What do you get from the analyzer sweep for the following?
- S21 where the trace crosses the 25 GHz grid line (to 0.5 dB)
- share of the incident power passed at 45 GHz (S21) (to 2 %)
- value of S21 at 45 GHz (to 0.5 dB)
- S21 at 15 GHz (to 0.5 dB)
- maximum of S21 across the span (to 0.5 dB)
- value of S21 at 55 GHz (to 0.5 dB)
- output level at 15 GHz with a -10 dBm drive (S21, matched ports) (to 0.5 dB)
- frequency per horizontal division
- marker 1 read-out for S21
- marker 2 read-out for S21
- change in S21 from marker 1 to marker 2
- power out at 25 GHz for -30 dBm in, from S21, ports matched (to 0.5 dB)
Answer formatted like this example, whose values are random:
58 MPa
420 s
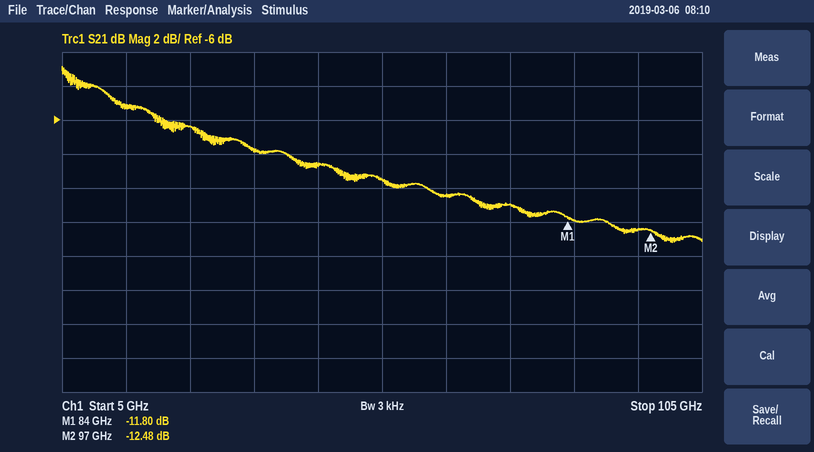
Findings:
-6.5 dB
14 %
-8.5 dB
-5.0 dB
-3.0 dB
-9.5 dB
-15.0 dBm
10 GHz
-11.80 dB
-12.48 dB
-0.68 dB
-36.5 dBm
